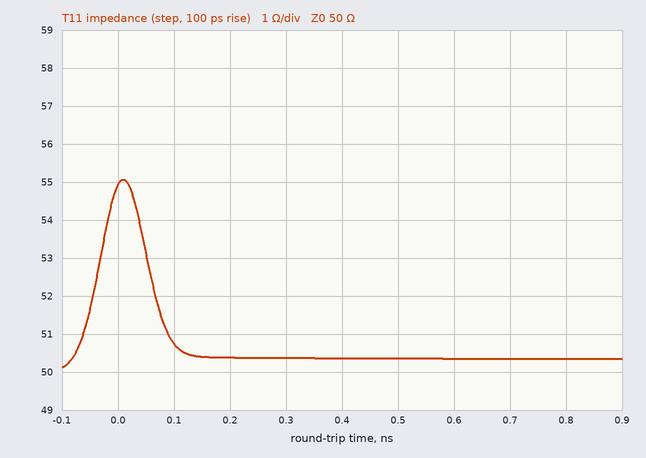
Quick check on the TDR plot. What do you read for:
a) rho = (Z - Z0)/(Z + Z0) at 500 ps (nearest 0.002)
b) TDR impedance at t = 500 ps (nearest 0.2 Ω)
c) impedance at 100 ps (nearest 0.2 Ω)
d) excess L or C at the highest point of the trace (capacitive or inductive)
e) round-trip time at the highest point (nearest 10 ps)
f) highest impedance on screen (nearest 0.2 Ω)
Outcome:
+0.004
50.4 Ω
50.8 Ω
inductive
10 ps
55.0 Ω
